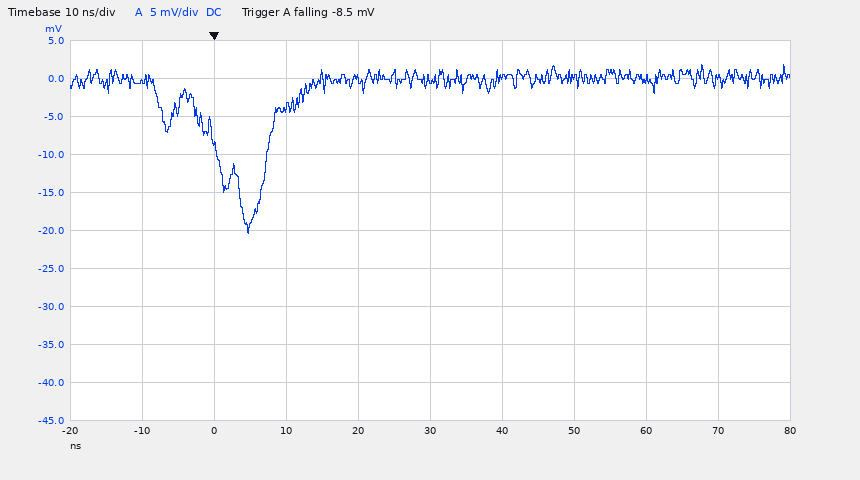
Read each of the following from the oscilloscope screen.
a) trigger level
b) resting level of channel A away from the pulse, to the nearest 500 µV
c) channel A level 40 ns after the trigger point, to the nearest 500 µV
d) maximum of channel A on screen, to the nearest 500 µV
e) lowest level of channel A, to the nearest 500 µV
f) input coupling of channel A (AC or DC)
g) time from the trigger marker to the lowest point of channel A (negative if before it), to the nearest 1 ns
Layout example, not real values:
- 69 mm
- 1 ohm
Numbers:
- -8.5 mV
- 0.0 mV
- 0.0 mV
- 2.0 mV
- -20.5 mV
- DC
- +5 ns
